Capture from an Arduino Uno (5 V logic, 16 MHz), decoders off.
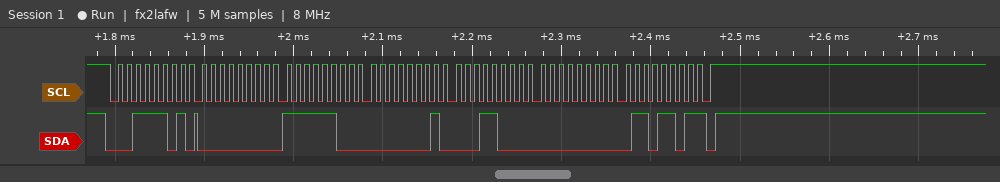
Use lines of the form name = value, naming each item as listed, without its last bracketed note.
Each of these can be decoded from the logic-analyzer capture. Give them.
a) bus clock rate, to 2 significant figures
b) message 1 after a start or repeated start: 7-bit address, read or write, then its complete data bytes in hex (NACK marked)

bus clock rate, to 2 significant figures = 100 kHz
message 1 after a start or repeated start: 7-bit address, read or write, then its complete data bytes in hex = 0x1E read: 00 FC 01 18 00 6D NACK
